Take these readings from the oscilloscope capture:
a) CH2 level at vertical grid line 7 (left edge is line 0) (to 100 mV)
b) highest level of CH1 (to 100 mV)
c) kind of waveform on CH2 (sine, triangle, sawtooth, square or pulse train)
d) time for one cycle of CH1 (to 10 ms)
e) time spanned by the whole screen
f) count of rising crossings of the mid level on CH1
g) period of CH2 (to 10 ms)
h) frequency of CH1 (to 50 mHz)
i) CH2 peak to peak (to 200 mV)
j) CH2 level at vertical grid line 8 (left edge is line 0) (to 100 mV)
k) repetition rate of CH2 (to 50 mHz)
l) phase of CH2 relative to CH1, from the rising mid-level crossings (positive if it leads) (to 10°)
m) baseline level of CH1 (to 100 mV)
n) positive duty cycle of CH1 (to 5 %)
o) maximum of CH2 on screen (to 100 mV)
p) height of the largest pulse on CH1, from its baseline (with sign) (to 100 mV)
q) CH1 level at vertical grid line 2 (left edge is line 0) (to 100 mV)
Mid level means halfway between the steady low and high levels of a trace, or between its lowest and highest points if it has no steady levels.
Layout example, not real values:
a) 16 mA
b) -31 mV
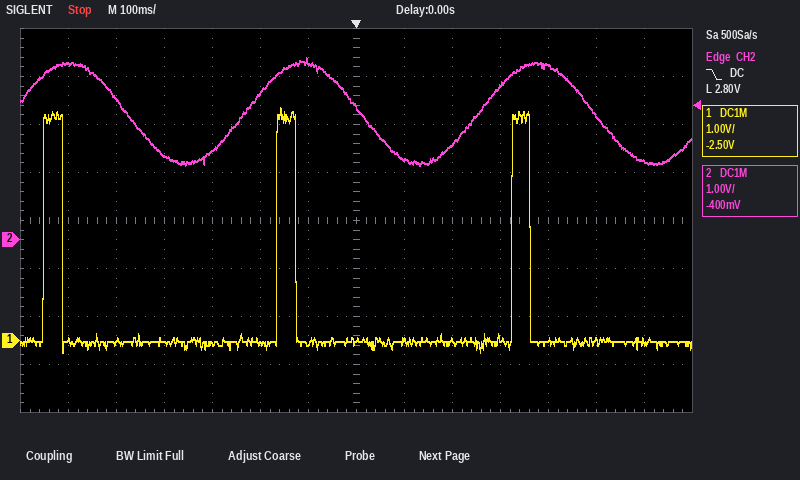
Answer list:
a) 2.8 V
b) 4.9 V
c) sine
d) 490 ms
e) 1.4 s
f) 3
g) 490 ms
h) 2.05 Hz
i) 2.2 V
j) 1.7 V
k) 2.05 Hz
l) +50°
m) 0.0 V
n) 10 %
o) 3.8 V
p) +4.9 V
q) 0.0 V
